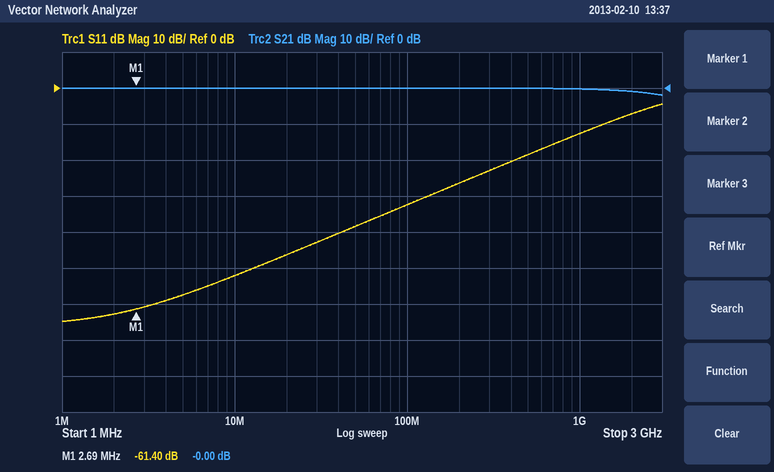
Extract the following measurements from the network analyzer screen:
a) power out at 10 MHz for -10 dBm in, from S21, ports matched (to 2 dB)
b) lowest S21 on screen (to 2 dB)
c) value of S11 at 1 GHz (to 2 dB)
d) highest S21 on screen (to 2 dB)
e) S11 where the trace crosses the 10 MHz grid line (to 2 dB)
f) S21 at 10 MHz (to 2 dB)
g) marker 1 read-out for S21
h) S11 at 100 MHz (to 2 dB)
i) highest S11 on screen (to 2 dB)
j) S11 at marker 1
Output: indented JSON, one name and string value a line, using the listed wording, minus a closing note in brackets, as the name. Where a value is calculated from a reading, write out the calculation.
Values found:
{
  "power out at 10 MHz for -10 dBm in, from S21, ports matched": "-10 dBm + (0 dB) = -10 dBm",
  "lowest S21 on screen": "-2 dB",
  "value of S11 at 1 GHz": "-12 dB",
  "highest S21 on screen": "0 dB",
  "S11 where the trace crosses the 10 MHz grid line": "-52 dB",
  "S21 at 10 MHz": "0 dB",
  "marker 1 read-out for S21": "-0.00 dB",
  "S11 at 100 MHz": "-32 dB",
  "highest S11 on screen": "-4 dB",
  "S11 at marker 1": "-61.40 dB"
}
